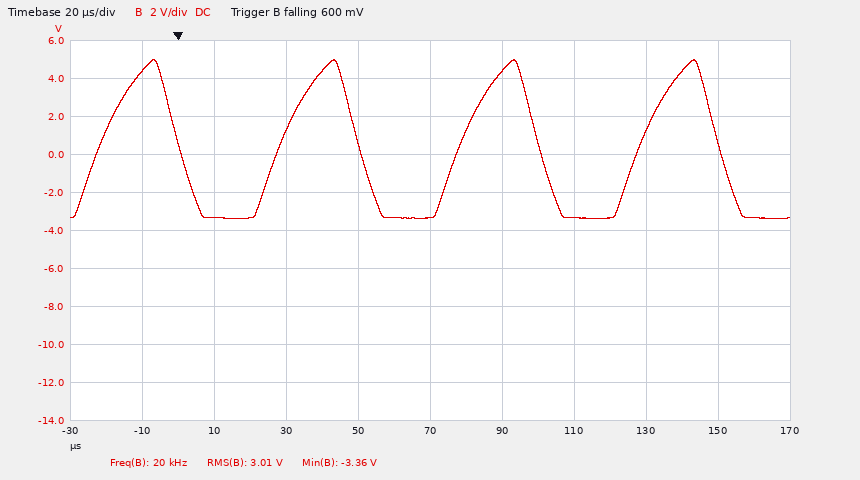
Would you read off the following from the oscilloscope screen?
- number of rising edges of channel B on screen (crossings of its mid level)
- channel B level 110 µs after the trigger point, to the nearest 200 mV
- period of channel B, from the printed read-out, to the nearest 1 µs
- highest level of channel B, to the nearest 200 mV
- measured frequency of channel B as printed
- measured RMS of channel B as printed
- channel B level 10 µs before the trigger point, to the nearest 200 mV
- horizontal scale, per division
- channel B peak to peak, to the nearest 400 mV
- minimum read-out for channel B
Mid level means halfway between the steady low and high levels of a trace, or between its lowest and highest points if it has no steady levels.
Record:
4
-3.4 V
50 µs
5.0 V
20 kHz
3.01 V
4.4 V
20 µs
8.4 V
-3.36 V
